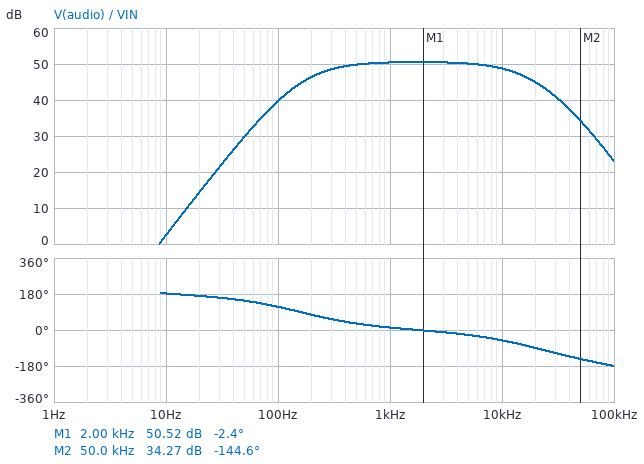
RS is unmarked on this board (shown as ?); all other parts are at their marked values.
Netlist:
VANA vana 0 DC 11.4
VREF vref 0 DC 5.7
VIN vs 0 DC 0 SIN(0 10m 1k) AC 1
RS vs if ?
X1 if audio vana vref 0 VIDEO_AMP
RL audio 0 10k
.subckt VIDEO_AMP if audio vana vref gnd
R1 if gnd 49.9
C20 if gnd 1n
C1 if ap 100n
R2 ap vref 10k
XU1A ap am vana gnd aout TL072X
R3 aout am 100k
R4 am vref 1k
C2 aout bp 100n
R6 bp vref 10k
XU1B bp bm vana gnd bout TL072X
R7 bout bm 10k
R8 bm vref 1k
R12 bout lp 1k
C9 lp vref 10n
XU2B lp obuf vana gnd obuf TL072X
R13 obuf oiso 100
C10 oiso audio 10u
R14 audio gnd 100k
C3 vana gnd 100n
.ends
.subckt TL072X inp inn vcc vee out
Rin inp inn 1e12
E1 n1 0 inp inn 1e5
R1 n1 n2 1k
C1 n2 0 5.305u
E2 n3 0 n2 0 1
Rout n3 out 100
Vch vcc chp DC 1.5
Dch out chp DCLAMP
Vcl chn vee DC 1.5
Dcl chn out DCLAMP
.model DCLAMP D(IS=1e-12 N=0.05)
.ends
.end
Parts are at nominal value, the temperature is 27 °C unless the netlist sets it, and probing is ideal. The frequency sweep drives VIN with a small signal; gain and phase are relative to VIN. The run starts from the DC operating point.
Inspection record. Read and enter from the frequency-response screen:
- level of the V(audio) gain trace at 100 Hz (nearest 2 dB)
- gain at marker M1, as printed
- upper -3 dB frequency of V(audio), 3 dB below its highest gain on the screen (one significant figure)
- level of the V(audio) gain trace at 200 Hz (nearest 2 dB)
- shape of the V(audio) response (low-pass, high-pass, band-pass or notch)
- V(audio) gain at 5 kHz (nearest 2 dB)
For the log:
40 dB
50.52 dB
10 kHz
46 dB
band-pass
50 dB
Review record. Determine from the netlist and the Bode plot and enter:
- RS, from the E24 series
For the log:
110 Ω
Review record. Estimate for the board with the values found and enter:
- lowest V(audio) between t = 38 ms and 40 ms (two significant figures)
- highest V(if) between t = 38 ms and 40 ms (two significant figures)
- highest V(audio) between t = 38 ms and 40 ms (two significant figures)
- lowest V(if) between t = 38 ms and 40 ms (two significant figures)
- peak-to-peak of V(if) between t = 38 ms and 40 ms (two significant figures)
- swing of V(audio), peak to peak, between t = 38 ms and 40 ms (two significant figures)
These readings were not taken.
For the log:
-3.3 V
3.1 mV
3.3 V
-3.1 mV
6.2 mV
6.6 V
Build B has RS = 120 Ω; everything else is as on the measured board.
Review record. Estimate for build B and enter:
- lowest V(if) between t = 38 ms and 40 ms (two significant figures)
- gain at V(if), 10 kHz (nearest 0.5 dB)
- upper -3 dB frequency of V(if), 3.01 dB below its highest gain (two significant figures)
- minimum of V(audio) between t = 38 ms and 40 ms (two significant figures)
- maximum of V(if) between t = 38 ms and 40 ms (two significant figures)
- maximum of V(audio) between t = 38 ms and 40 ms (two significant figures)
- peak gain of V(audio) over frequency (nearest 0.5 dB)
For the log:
-2.9 mV
-10.5 dB
4.5 MHz
-3.1 V
2.9 mV
3.1 V
50.0 dB
